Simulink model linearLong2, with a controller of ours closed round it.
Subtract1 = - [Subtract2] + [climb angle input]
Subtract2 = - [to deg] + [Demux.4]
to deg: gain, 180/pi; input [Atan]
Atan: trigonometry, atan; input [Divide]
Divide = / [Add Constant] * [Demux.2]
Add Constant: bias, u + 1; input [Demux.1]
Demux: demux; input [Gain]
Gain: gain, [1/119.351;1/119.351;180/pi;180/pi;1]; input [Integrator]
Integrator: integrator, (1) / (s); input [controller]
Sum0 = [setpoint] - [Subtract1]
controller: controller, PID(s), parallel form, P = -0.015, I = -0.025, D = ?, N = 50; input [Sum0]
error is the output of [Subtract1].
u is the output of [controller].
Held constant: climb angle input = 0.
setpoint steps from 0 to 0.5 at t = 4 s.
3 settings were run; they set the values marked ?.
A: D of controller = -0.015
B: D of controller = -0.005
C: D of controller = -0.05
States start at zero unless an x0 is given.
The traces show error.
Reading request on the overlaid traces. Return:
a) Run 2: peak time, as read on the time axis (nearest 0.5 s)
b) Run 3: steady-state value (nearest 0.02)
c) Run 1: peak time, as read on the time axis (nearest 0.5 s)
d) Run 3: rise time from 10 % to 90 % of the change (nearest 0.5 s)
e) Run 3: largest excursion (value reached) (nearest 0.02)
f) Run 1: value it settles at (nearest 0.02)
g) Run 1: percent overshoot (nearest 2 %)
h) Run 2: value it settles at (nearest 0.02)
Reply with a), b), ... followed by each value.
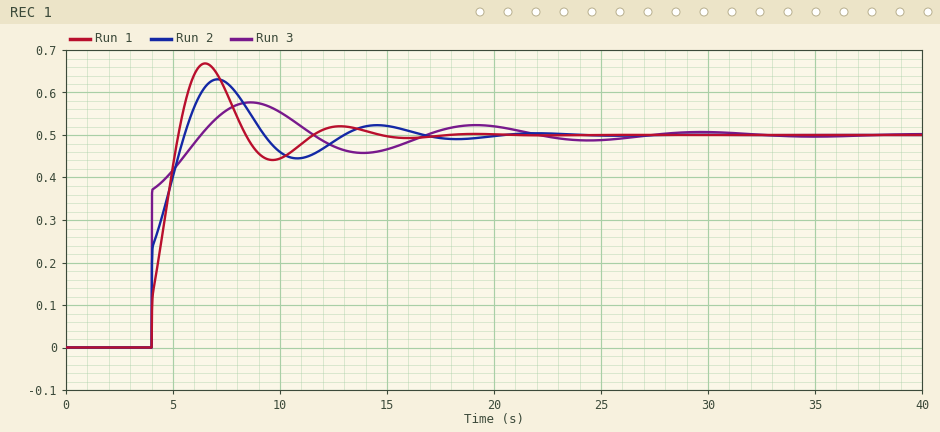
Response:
a) 7.0 s
b) 0.50
c) 6.5 s
d) 1.5 s
e) 0.58
f) 0.50
g) 34 %
h) 0.50
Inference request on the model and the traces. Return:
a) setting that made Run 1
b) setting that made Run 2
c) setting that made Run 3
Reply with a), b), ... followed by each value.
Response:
a) B
b) A
c) C
